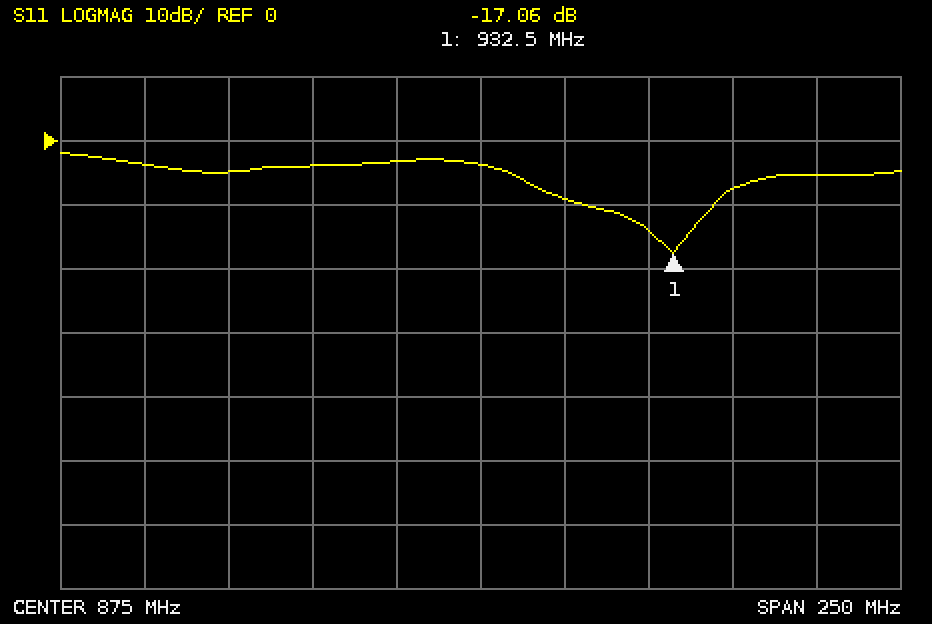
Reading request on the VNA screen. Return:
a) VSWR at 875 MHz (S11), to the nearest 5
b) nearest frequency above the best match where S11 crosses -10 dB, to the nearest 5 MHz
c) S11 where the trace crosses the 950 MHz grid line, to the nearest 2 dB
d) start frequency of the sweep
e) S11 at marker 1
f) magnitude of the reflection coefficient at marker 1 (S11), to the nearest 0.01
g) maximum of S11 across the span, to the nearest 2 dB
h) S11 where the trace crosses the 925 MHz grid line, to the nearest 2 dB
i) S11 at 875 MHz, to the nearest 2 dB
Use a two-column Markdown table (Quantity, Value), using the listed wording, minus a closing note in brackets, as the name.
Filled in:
| Quantity | Value |
|---|---|
| VSWR at 875 MHz (S11), to the nearest 5 | 5 |
| nearest frequency above the best match where S11 crosses -10 dB, to the nearest 5 MHz | 945 MHz |
| S11 where the trace crosses the 950 MHz grid line, to the nearest 2 dB | -8 dB |
| start frequency of the sweep | 750 MHz |
| S11 at marker 1 | -17.06 dB |
| magnitude of the reflection coefficient at marker 1 (S11), to the nearest 0.01 | 0.14 |
| maximum of S11 across the span, to the nearest 2 dB | -2 dB |
| S11 where the trace crosses the 925 MHz grid line, to the nearest 2 dB | -14 dB |
| S11 at 875 MHz, to the nearest 2 dB | -4 dB |
